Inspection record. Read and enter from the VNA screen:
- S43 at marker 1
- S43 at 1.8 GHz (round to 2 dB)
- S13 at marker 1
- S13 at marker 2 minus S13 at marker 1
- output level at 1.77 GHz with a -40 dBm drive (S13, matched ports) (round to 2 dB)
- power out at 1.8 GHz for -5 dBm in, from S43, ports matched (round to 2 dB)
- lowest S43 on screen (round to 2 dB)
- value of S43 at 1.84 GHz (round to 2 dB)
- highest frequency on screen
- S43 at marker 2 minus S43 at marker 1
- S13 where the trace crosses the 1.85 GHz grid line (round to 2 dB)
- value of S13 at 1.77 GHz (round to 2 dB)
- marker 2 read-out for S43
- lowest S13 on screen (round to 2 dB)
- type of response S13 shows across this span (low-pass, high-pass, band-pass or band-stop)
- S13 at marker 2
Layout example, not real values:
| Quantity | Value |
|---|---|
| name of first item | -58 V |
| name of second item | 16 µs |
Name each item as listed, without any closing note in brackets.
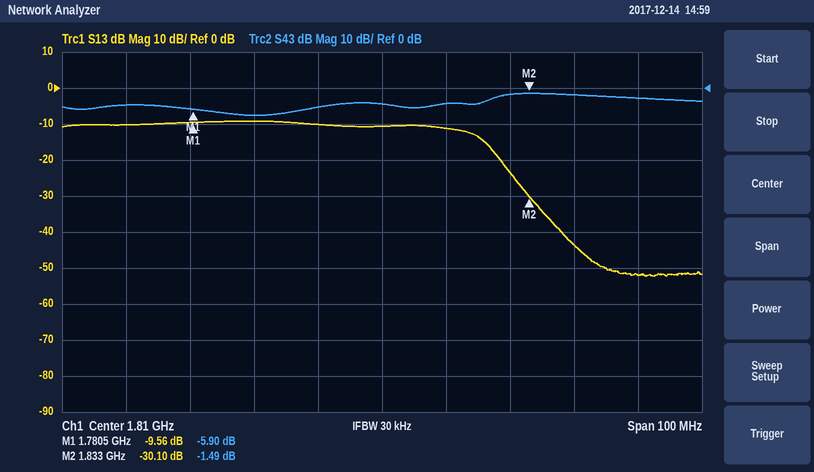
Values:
| Quantity | Value |
|---|---|
| S43 at marker 1 | -5.90 dB |
| S43 at 1.8 GHz | -6 dB |
| S13 at marker 1 | -9.56 dB |
| S13 at marker 2 minus S13 at marker 1 | -20.54 dB |
| output level at 1.77 GHz with a -40 dBm drive (S13, matched ports) | -50 dBm |
| power out at 1.8 GHz for -5 dBm in, from S43, ports matched | -10 dBm |
| lowest S43 on screen | -8 dB |
| value of S43 at 1.84 GHz | -2 dB |
| highest frequency on screen | 1.86 GHz |
| S43 at marker 2 minus S43 at marker 1 | 4.41 dB |
| S13 where the trace crosses the 1.85 GHz grid line | -52 dB |
| value of S13 at 1.77 GHz | -10 dB |
| marker 2 read-out for S43 | -1.49 dB |
| lowest S13 on screen | -52 dB |
| type of response S13 shows across this span | low-pass |
| S13 at marker 2 | -30.10 dB |
